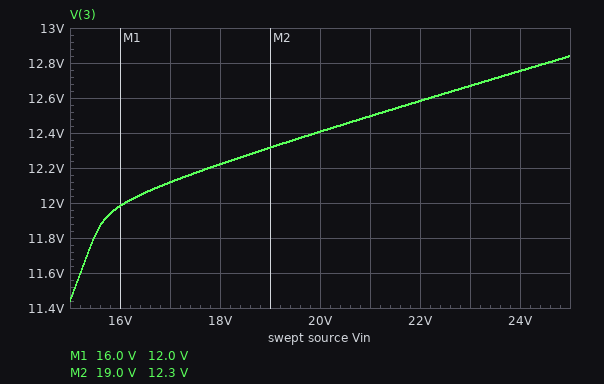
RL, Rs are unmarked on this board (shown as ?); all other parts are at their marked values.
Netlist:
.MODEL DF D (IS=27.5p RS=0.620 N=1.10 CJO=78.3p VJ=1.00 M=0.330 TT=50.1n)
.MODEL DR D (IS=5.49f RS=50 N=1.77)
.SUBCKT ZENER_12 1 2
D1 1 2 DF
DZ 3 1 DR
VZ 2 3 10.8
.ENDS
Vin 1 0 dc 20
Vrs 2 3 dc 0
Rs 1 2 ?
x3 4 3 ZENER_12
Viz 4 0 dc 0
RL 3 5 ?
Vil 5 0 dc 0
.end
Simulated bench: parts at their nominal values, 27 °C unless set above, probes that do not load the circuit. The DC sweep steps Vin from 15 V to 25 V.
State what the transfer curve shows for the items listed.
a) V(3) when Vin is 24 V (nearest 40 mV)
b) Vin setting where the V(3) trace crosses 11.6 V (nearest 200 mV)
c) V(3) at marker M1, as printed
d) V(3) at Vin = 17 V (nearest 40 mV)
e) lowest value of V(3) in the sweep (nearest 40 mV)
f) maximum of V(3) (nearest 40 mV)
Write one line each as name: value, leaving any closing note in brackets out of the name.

V(3) when Vin is 24 V: 12.76 V
Vin setting where the V(3) trace crosses 11.6 V: 15.2 V
V(3) at marker M1, as printed: 12.0 V
V(3) at Vin = 17 V: 12.12 V
lowest value of V(3) in the sweep: 11.44 V
maximum of V(3): 12.84 V
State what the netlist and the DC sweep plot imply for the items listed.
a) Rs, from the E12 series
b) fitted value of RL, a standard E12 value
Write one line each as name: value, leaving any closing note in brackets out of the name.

Rs, from the E12 series: 560 Ω
fitted value of RL, a standard E12 value: 1.8 kΩ
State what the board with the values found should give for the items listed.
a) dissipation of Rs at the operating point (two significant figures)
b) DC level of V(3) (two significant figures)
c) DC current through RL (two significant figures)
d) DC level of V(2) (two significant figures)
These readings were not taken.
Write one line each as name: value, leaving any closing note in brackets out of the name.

dissipation of Rs at the operating point: 100 mW
DC level of V(3): 12 V
DC current through RL: 6.9 mA
DC level of V(2): 12 V
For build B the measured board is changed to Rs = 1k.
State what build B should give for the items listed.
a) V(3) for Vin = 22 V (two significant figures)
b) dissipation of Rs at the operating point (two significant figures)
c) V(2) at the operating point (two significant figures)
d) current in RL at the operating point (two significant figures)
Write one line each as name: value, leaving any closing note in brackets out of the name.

V(3) for Vin = 22 V: 12 V
dissipation of Rs at the operating point: 63 mW
V(2) at the operating point: 12 V
current in RL at the operating point: 6.7 mA
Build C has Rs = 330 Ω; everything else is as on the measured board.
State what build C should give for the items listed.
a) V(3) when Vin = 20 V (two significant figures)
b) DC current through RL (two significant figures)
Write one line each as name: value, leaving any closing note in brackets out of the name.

V(3) when Vin = 20 V: 13 V
DC current through RL: 7.1 mA
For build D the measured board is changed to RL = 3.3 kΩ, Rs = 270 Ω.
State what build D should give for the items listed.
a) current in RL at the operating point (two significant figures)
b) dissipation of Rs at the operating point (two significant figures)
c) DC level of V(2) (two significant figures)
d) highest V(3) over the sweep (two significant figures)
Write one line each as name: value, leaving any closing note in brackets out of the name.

current in RL at the operating point: 4.0 mA
dissipation of Rs at the operating point: 170 mW
DC level of V(2): 13 V
highest V(3) over the sweep: 14 V
